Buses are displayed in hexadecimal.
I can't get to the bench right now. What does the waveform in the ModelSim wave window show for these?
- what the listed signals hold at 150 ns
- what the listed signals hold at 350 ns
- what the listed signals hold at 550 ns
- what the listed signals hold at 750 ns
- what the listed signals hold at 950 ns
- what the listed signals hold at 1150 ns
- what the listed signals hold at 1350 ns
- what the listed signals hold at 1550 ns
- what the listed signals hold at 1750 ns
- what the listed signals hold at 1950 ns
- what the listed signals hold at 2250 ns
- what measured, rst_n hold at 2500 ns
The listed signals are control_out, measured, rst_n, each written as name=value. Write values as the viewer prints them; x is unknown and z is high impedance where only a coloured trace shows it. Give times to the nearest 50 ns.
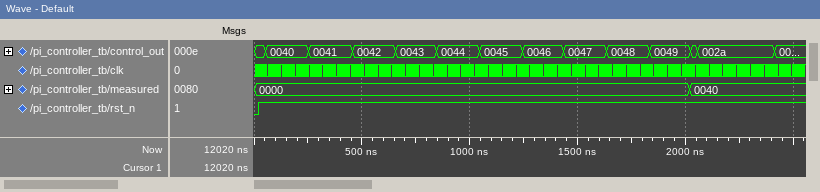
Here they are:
control_out=0040, measured=0000, rst_n=1
control_out=0041, measured=0000, rst_n=1
control_out=0042, measured=0000, rst_n=1
control_out=0043, measured=0000, rst_n=1
control_out=0044, measured=0000, rst_n=1
control_out=0045, measured=0000, rst_n=1
control_out=0046, measured=0000, rst_n=1
control_out=0047, measured=0000, rst_n=1
control_out=0048, measured=0000, rst_n=1
control_out=0049, measured=0000, rst_n=1
control_out=002a, measured=0040, rst_n=1
measured=0040, rst_n=1
